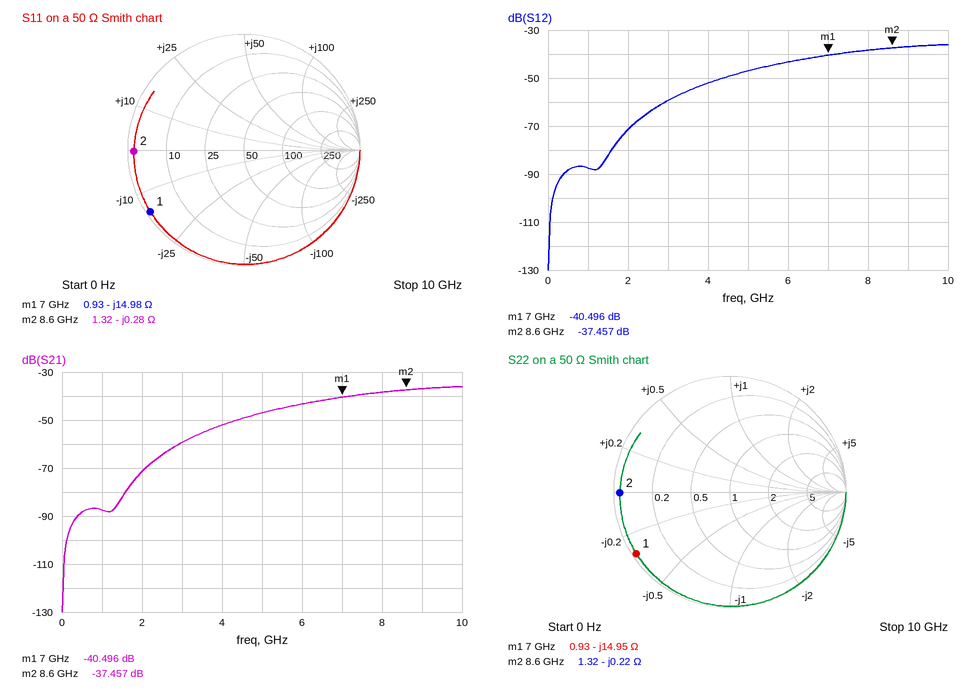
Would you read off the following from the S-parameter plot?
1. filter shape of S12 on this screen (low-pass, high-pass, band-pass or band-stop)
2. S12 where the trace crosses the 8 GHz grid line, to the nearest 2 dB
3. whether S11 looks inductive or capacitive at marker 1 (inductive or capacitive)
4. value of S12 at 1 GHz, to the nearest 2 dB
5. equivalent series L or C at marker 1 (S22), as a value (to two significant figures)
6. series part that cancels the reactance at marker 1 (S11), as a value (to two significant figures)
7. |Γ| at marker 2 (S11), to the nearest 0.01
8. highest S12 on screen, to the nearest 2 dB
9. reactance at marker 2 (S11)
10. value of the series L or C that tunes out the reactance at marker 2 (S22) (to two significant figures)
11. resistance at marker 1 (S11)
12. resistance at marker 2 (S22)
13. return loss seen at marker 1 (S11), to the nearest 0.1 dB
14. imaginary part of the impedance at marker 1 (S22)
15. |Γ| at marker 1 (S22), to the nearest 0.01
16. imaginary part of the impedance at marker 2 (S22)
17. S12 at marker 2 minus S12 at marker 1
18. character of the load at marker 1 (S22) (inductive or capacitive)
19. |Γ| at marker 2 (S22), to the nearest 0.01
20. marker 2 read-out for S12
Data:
high-pass
-38 dB
capacitive
-88 dB
1.5 pF
340 pH
0.95
-36 dB
-0.28 Ω
4.1 pH
0.93 Ω
1.32 Ω
0.3 dB
-14.95 Ω
0.97
-0.22 Ω
3.039 dB
capacitive
0.95
-37.457 dB
